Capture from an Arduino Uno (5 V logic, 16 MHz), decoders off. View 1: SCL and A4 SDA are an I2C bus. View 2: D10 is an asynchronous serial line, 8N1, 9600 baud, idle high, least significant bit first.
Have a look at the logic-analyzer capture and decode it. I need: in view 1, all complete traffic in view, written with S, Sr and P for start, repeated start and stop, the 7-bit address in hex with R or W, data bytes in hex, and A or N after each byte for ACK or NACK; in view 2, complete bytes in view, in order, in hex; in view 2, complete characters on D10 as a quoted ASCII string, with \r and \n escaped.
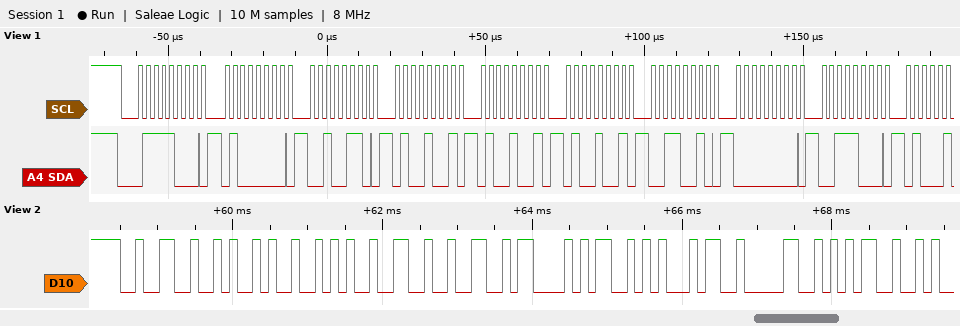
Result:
S 3CW A 40 A 26 A 49 A 49 A 49 A 32 A 00 A 38 A
32 4A 52 32 32 43 53 34 30 35
"2JR22CS405"
